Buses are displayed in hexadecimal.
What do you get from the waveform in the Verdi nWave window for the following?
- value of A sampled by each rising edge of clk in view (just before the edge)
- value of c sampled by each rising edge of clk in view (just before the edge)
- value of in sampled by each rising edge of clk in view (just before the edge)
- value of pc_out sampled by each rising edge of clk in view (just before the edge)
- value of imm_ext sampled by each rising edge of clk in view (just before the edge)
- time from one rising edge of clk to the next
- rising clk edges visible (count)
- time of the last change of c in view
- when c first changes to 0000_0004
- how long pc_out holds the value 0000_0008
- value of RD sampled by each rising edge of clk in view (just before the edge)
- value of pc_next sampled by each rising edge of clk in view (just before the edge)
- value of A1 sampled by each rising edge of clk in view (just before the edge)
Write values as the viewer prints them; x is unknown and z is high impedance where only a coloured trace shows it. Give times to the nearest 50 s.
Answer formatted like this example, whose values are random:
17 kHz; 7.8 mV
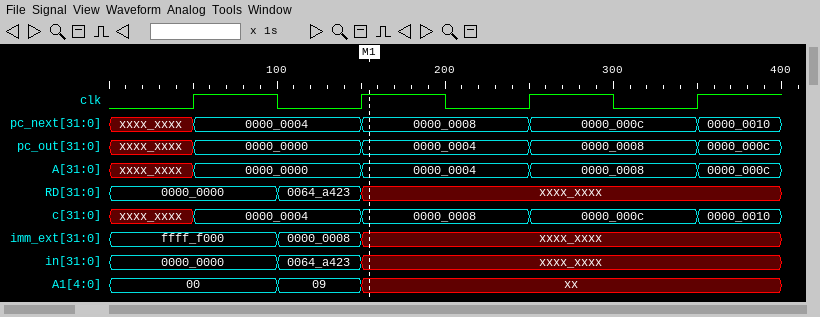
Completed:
xxxx_xxxx, 0000_0000, 0000_0004, 0000_0008; xxxx_xxxx, 0000_0004, 0000_0008, 0000_000c; 0000_0000, 0064_a423, xxxx_xxxx, xxxx_xxxx; xxxx_xxxx, 0000_0000, 0000_0004, 0000_0008; ffff_f000, 0000_0008, xxxx_xxxx, xxxx_xxxx; 100 s; 4; 350 s; 50 s; 100 s; 0000_0000, 0064_a423, xxxx_xxxx, xxxx_xxxx; xxxx_xxxx, 0000_0004, 0000_0008, 0000_000c; 00, 09, xx, xx
